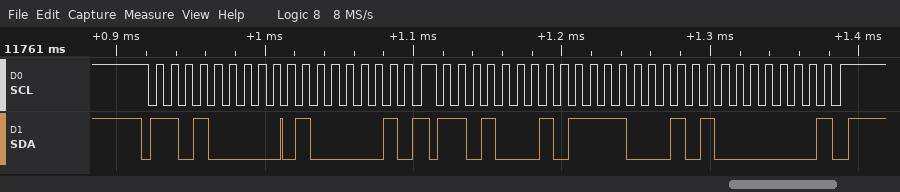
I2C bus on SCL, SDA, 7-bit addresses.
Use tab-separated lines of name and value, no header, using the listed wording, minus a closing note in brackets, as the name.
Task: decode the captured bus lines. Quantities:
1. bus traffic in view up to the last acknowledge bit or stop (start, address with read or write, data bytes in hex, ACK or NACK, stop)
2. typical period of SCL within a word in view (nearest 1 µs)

bus traffic in view up to the last acknowledge bit or stop	start, address 68 write ACK, 41 ACK, repeated start, address 68 read ACK, F1 ACK, 80 NACK, stop
typical period of SCL within a word in view	10 µs
